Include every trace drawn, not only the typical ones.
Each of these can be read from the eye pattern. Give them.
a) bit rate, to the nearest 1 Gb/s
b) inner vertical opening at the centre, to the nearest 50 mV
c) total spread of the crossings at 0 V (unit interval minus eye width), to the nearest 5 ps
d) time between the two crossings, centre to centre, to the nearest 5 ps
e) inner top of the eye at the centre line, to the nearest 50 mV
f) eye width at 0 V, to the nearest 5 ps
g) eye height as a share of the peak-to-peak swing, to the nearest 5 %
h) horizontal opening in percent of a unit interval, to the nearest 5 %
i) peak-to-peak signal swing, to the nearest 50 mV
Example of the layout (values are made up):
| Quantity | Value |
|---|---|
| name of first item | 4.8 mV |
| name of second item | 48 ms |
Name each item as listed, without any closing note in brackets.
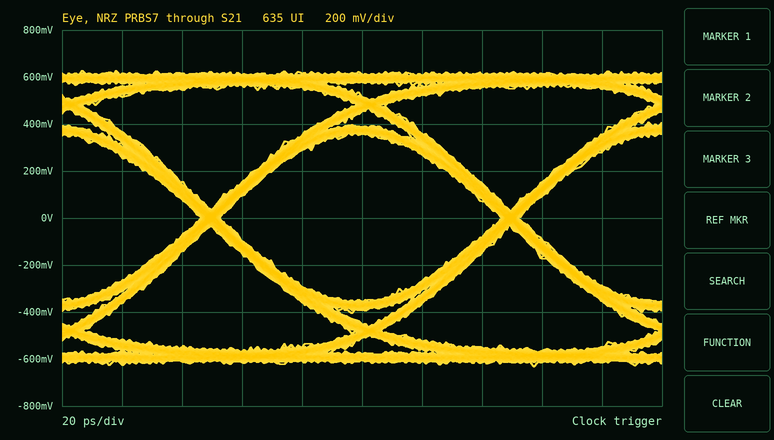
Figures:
| Quantity | Value |
|---|---|
| bit rate, to the nearest 1 Gb/s | 10 Gb/s |
| inner vertical opening at the centre, to the nearest 50 mV | 700 mV |
| total spread of the crossings at 0 V (unit interval minus eye width), to the nearest 5 ps | 5 ps |
| time between the two crossings, centre to centre, to the nearest 5 ps | 100 ps |
| inner top of the eye at the centre line, to the nearest 50 mV | 350 mV |
| eye width at 0 V, to the nearest 5 ps | 95 ps |
| eye height as a share of the peak-to-peak swing, to the nearest 5 % | 55 % |
| horizontal opening in percent of a unit interval, to the nearest 5 % | 95 % |
| peak-to-peak signal swing, to the nearest 50 mV | 1.25 V |
